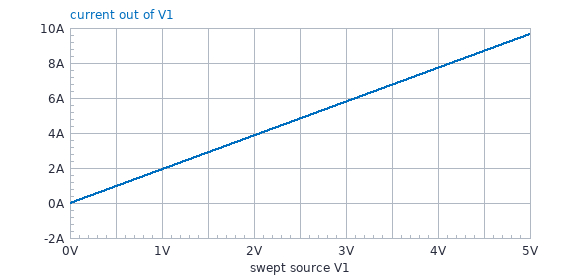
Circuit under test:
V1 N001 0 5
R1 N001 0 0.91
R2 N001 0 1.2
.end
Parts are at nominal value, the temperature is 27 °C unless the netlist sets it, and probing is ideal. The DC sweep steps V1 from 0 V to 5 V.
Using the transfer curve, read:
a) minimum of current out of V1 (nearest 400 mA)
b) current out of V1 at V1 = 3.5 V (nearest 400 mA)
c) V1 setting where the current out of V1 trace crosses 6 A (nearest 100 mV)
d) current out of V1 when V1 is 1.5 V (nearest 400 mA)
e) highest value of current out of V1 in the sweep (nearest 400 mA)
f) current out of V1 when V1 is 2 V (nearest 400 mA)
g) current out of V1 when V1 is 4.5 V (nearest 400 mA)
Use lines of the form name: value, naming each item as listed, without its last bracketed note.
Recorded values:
minimum of current out of V1: 0 A
current out of V1 at V1 = 3.5 V: 6.8 A
V1 setting where the current out of V1 trace crosses 6 A: 3.1 V
current out of V1 when V1 is 1.5 V: 2.8 A
highest value of current out of V1 in the sweep: 9.6 A
current out of V1 when V1 is 2 V: 4.0 A
current out of V1 when V1 is 4.5 V: 8.8 A
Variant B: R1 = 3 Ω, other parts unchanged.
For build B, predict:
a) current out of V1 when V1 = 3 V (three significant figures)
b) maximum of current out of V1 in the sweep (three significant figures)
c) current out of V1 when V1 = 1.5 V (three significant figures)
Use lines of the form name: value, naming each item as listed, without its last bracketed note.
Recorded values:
current out of V1 when V1 = 3 V: 3.50 A
maximum of current out of V1 in the sweep: 5.83 A
current out of V1 when V1 = 1.5 V: 1.75 A
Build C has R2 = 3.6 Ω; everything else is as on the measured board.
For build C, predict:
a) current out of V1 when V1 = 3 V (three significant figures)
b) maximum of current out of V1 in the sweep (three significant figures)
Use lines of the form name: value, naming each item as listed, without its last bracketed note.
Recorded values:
current out of V1 when V1 = 3 V: 4.13 A
maximum of current out of V1 in the sweep: 6.88 A
